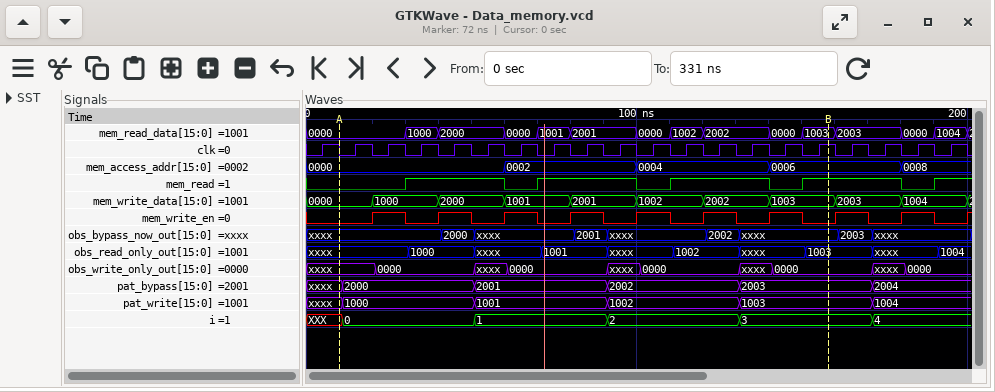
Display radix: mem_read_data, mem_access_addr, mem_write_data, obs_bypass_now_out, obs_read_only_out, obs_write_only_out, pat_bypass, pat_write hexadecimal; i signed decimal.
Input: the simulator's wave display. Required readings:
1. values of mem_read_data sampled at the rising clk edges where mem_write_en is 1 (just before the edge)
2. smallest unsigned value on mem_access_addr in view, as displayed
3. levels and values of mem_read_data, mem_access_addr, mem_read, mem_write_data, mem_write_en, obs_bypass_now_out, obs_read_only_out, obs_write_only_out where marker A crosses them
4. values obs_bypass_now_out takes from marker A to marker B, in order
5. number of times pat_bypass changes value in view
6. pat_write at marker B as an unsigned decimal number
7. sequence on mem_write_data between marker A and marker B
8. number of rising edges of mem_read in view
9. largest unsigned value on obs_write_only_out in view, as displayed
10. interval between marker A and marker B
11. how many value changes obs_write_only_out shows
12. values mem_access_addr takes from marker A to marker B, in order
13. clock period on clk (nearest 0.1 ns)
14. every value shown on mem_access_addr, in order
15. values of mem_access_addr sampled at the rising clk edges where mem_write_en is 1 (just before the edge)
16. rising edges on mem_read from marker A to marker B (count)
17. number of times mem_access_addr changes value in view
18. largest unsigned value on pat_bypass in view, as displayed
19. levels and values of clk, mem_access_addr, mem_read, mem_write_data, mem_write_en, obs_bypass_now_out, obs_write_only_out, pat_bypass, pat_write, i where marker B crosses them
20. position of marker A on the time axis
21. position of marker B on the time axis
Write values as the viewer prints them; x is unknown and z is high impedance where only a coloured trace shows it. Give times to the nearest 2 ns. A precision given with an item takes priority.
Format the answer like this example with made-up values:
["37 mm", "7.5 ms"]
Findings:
["0000, 2000, 0000, 2001, 0000, 2002, 0000, 2003, 0000", "0000", "mem_read_data=0000, mem_access_addr=0000, mem_read=0, mem_write_data=0000, mem_write_en=0, obs_bypass_now_out=xxxx, obs_read_only_out=xxxx, obs_write_only_out=xxxx", "xxxx, 2000, xxxx, 2001, xxxx, 2002, xxxx", "5", "4099", "0000, 1000, 2000, 1001, 2001, 1002, 2002, 1003", "5", "0000", "148 ns", "9", "0000, 0002, 0004, 0006", "10 ns", "0000, 0002, 0004, 0006, 0008", "0000, 0000, 0002, 0002, 0004, 0004, 0006, 0006, 0008", "4", "4", "2004", "clk=1, mem_access_addr=0006, mem_read=1, mem_write_data=1003, mem_write_en=0, obs_bypass_now_out=xxxx, obs_write_only_out=0000, pat_bypass=2003, pat_write=1003, i=3", "10 ns", "158 ns"]
